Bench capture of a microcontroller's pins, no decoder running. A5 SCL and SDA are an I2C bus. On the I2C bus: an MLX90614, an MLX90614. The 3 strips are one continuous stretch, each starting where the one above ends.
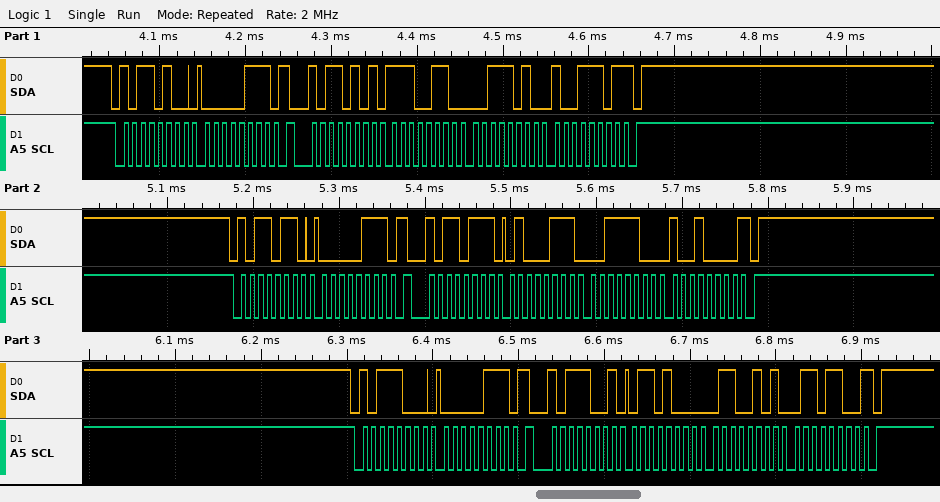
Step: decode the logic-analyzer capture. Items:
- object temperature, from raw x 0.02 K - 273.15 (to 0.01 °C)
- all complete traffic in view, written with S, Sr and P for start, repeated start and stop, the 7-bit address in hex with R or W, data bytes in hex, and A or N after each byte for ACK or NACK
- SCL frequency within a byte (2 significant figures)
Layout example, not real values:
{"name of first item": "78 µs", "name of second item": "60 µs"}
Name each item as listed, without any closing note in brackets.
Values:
{"object temperature, from raw x 0.02 K - 273.15": "28.41 °C", "all complete traffic in view, written with S, Sr and P for start, repeated start and stop, the 7-bit address in hex with R or W, data bytes in hex, and A or N after each byte for ACK or NACK": "S 5AW A 07 A Sr 5AR A E6 A 3A A 9D N P S 5BW A 07 A Sr 5BR A 47 A 3C A 90 N P S 5CW A 07 A Sr 5CR A 68 A 65 A 6C N P", "SCL frequency within a byte": "100 kHz"}
